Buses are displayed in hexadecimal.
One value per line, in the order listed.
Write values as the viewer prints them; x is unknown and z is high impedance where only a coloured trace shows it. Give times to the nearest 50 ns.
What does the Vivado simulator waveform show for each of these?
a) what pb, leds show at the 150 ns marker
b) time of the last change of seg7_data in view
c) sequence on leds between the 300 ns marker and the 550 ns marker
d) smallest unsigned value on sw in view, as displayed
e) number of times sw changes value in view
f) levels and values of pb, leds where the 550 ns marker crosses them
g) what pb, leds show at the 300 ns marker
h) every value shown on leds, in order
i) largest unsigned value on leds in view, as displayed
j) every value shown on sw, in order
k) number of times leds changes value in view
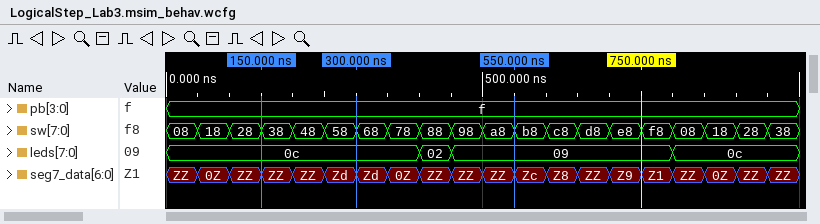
pb=f, leds=0c
950 ns
0c, 02, 09
08
19
pb=f, leds=09
pb=f, leds=0c
0c, 02, 09, 0c
0c
08, 18, 28, 38, 48, 58, 68, 78, 88, 98, a8, b8, c8, d8, e8, f8, 08, 18, 28, 38
3
